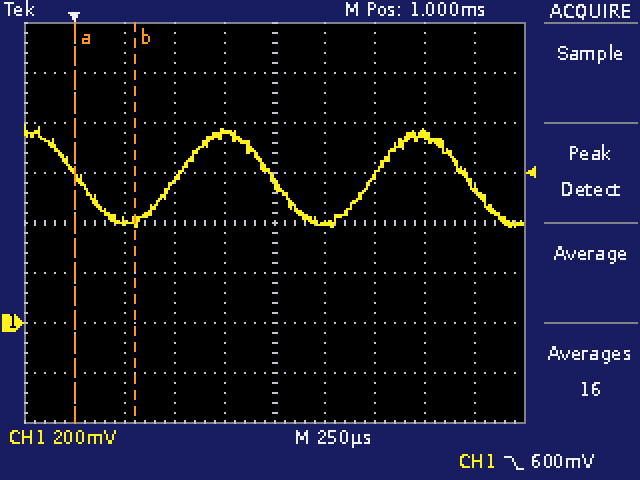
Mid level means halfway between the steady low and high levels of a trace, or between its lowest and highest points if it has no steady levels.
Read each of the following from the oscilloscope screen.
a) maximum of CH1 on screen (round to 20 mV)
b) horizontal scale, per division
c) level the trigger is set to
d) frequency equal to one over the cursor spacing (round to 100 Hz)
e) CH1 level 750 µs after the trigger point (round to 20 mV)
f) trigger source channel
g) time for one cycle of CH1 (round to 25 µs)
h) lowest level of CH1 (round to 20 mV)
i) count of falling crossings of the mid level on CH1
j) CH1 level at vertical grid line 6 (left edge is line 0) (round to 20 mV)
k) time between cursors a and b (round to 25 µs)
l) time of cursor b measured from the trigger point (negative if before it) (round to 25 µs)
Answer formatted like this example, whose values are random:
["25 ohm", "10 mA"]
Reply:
["800 mV", "250 µs", "600 mV", "3.3 kHz", "760 mV", "CH1", "975 µs", "380 mV", "3", "400 mV", "300 µs", "+300 µs"]
